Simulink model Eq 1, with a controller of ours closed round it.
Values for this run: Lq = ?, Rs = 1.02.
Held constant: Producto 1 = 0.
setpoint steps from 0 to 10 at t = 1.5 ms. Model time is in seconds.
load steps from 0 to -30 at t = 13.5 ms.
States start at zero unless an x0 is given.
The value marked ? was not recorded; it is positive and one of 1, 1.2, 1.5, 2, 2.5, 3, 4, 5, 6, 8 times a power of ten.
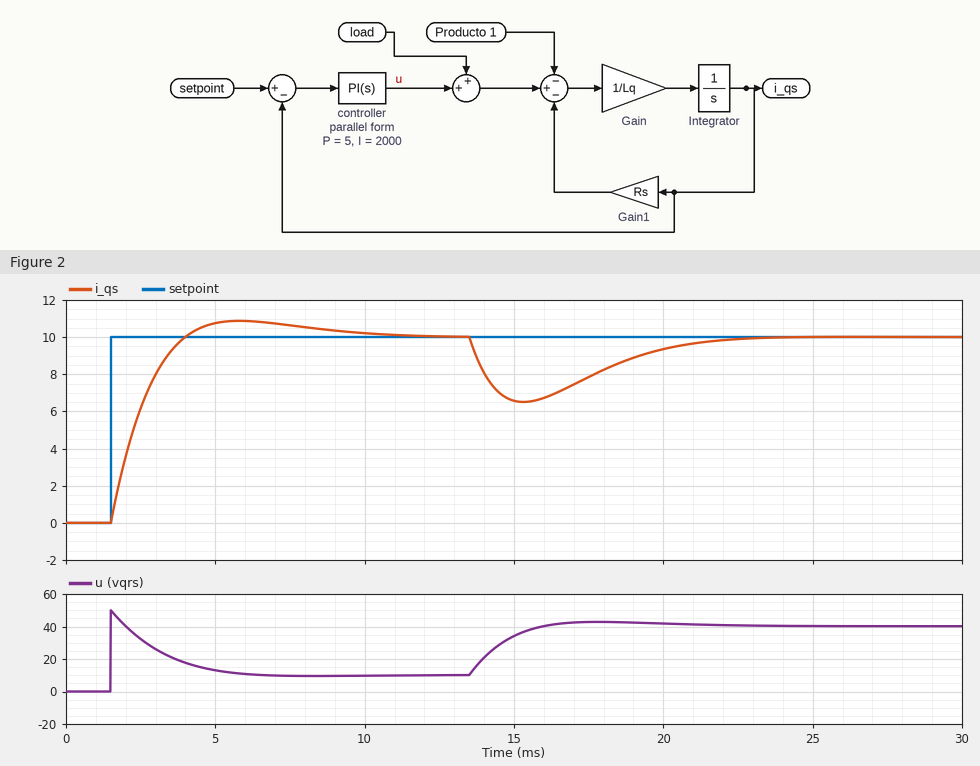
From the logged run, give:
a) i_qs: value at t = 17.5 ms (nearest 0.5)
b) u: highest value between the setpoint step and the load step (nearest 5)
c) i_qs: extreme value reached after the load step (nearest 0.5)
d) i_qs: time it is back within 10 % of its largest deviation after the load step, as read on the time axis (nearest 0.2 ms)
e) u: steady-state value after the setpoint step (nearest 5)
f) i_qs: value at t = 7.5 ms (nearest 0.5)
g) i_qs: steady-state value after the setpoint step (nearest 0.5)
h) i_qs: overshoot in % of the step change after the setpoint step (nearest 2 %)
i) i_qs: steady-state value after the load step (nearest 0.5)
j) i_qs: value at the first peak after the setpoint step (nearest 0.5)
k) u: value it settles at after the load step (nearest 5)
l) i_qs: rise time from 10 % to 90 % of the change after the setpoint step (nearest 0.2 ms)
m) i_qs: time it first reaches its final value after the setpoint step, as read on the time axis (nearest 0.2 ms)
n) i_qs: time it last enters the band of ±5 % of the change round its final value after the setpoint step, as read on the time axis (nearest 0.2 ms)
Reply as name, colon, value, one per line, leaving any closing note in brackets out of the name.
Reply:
i_qs: value at t = 17.5 ms: 8.0
u: highest value between the setpoint step and the load step: 50
i_qs: extreme value reached after the load step: 6.5
i_qs: time it is back within 10 % of its largest deviation after the load step, as read on the time axis: 21.0 ms
u: steady-state value after the setpoint step: 10
i_qs: value at t = 7.5 ms: 10.5
i_qs: steady-state value after the setpoint step: 10.0
i_qs: overshoot in % of the step change after the setpoint step: 8 %
i_qs: steady-state value after the load step: 10.0
i_qs: value at the first peak after the setpoint step: 11.0
u: value it settles at after the load step: 40
i_qs: rise time from 10 % to 90 % of the change after the setpoint step: 1.8 ms
i_qs: time it first reaches its final value after the setpoint step, as read on the time axis: 4.0 ms
i_qs: time it last enters the band of ±5 % of the change round its final value after the setpoint step, as read on the time axis: 8.2 ms
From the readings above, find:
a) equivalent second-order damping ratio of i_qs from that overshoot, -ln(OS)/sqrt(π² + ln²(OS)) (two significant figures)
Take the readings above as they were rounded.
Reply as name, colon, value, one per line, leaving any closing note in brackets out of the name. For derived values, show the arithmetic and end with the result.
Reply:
equivalent second-order damping ratio of i_qs from that overshoot, -ln(OS)/sqrt(π² + ln²(OS)): ln(0.08) = -2.526; 2.526 / sqrt(9.870 + 6.379) = 0.63
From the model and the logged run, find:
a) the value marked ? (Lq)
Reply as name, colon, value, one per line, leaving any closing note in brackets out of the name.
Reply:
the value marked ?: 0.006
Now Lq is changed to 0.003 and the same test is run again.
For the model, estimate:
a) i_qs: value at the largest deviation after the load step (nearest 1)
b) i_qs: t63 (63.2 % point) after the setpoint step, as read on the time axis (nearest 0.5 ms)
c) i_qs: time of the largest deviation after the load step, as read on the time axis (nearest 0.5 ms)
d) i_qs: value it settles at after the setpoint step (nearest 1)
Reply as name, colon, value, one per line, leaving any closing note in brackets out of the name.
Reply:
i_qs: value at the largest deviation after the load step: 6
i_qs: t63 (63.2 % point) after the setpoint step, as read on the time axis: 2.0 ms
i_qs: time of the largest deviation after the load step, as read on the time axis: 14.5 ms
i_qs: value it settles at after the setpoint step: 10
